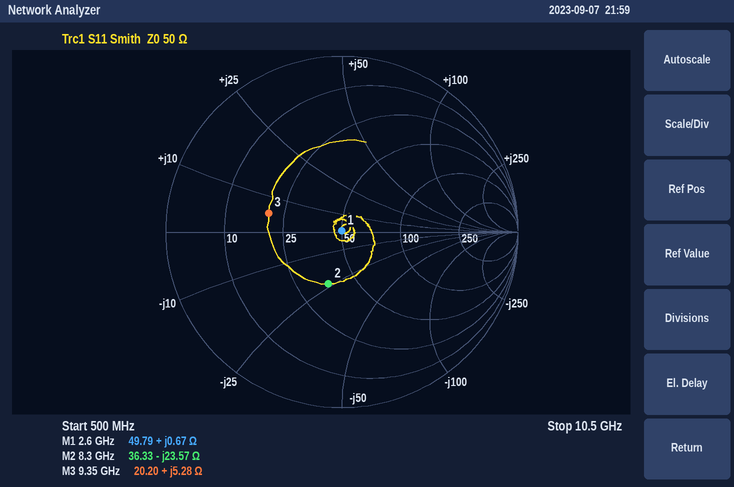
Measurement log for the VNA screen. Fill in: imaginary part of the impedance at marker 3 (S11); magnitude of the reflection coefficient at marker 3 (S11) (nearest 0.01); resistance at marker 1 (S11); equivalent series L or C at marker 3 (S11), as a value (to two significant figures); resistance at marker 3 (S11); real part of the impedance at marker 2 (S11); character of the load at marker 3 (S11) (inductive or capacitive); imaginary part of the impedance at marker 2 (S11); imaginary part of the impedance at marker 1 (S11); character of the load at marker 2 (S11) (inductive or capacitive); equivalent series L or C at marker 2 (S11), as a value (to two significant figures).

+5.28 Ω
0.43
49.79 Ω
90 pH
20.20 Ω
36.33 Ω
inductive
-23.57 Ω
+0.67 Ω
capacitive
810 fF
